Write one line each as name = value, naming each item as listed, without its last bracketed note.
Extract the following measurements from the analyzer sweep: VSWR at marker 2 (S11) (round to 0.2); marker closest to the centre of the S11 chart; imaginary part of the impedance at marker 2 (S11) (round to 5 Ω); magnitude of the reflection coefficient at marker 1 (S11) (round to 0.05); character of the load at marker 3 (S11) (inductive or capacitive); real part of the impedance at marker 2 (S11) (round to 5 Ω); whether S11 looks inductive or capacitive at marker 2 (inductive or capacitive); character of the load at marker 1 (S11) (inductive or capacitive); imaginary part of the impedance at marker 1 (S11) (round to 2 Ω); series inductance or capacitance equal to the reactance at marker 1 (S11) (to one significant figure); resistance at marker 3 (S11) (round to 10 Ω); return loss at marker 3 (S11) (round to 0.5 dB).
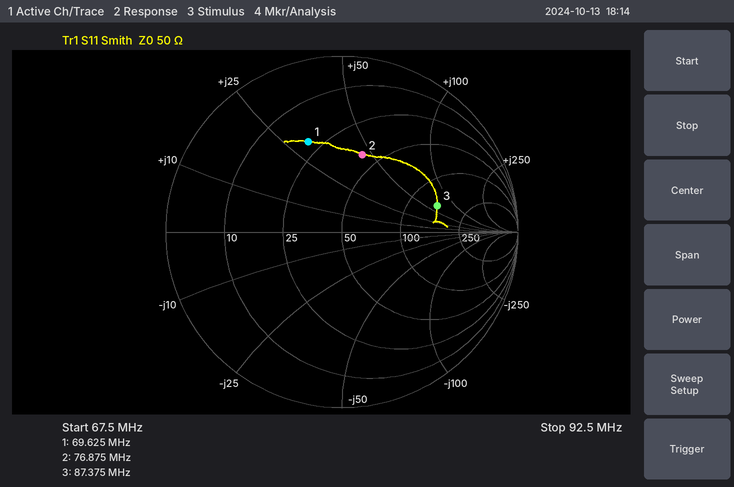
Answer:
VSWR at marker 2 (S11) = 2.6
marker closest to the centre of the S11 chart = marker 2
imaginary part of the impedance at marker 2 (S11) = +45 Ω
magnitude of the reflection coefficient at marker 1 (S11) = 0.55
character of the load at marker 3 (S11) = inductive
real part of the impedance at marker 2 (S11) = 40 Ω
whether S11 looks inductive or capacitive at marker 2 = inductive
character of the load at marker 1 (S11) = inductive
imaginary part of the impedance at marker 1 (S11) = +30 Ω
series inductance or capacitance equal to the reactance at marker 1 (S11) = 70 nH
resistance at marker 3 (S11) = 150 Ω
return loss at marker 3 (S11) = 5.0 dB
